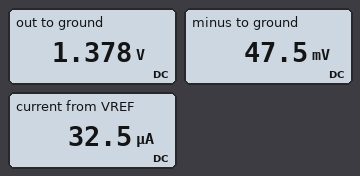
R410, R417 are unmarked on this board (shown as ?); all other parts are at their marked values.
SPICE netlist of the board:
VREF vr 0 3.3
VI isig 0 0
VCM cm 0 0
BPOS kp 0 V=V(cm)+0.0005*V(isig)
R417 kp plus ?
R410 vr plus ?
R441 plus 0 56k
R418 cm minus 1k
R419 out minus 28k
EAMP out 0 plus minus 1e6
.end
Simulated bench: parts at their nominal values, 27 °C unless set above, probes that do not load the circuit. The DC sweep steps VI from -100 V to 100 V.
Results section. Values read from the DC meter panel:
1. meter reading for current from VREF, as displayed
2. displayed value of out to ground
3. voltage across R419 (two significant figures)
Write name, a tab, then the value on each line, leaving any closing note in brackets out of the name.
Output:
meter reading for current from VREF, as displayed	32.5 µA
displayed value of out to ground	1.378 V
voltage across R419	1.3 V
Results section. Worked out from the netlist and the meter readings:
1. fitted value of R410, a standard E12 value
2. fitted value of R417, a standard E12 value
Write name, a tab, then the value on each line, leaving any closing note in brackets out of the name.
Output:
fitted value of R410, a standard E12 value	100 kΩ
fitted value of R417, a standard E12 value	1.5 kΩ
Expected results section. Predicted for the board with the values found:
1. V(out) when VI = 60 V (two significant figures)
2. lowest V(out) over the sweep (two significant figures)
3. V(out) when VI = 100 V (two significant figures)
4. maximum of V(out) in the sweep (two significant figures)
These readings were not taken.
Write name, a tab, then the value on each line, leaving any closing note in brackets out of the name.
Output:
V(out) when VI = 60 V	2.2 V
lowest V(out) over the sweep	-14 mV
V(out) when VI = 100 V	2.8 V
maximum of V(out) in the sweep	2.8 V
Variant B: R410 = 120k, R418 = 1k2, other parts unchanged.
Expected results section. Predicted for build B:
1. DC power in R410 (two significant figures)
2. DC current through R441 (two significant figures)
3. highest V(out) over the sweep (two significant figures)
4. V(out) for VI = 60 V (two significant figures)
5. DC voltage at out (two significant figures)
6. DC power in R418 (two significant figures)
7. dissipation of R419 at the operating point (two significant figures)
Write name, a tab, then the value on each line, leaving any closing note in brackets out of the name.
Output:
DC power in R410	89 µW
DC current through R441	710 nA
highest V(out) over the sweep	2.1 V
V(out) for VI = 60 V	1.7 V
DC voltage at out	970 mV
DC power in R418	1.3 µW
dissipation of R419 at the operating point	31 µW
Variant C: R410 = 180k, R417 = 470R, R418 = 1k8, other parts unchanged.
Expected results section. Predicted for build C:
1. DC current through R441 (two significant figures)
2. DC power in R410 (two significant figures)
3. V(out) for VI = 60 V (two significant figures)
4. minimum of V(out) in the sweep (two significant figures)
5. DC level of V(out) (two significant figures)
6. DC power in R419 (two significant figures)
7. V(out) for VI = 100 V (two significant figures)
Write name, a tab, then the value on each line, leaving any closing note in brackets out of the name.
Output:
DC current through R441	150 nA
DC power in R410	60 µW
V(out) for VI = 60 V	630 mV
minimum of V(out) in the sweep	-680 mV
DC level of V(out)	140 mV
DC power in R419	630 nW
V(out) for VI = 100 V	960 mV
